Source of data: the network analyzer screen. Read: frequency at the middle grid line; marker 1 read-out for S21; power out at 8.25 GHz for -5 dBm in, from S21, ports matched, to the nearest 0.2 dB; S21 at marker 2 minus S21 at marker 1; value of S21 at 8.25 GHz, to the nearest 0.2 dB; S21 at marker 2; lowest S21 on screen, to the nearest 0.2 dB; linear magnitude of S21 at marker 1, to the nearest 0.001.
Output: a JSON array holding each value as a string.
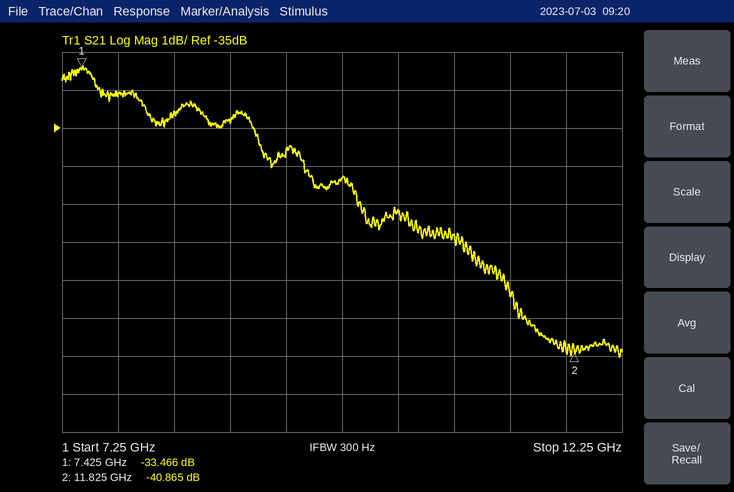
["9.75 GHz", "-33.466 dB", "-39.6 dBm", "-7.399 dB", "-34.6 dB", "-40.865 dB", "-41.0 dB", "0.021"]
